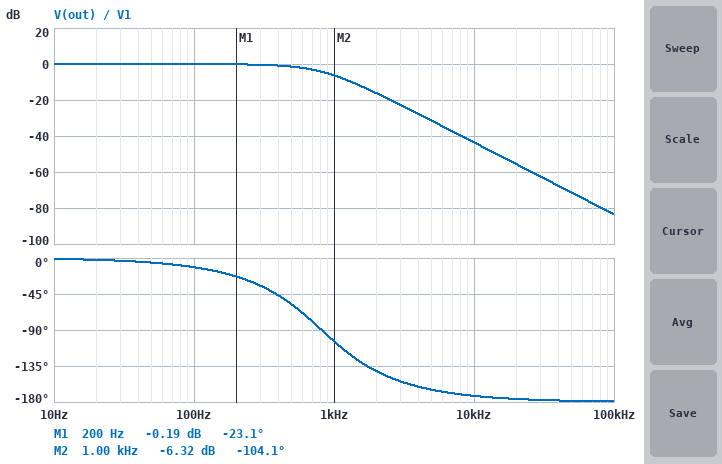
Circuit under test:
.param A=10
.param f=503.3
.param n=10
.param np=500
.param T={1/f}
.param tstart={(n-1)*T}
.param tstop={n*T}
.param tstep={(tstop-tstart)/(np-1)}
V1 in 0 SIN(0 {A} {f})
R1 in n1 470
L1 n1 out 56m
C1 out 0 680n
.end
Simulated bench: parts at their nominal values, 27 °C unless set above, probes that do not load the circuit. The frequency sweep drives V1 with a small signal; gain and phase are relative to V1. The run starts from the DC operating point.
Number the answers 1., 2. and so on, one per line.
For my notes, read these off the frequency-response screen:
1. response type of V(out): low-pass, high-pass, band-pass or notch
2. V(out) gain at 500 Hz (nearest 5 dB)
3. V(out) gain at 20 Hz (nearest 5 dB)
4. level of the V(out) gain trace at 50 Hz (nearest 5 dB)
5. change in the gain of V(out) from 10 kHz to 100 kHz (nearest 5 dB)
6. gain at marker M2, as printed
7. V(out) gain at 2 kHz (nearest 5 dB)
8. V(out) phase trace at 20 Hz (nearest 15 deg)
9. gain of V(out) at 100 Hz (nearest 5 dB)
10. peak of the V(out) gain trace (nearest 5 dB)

1. low-pass
2. 0 dB
3. 0 dB
4. 0 dB
5. -40 dB
6. -6.32 dB
7. -15 dB
8. 0 deg
9. 0 dB
10. 0 dB
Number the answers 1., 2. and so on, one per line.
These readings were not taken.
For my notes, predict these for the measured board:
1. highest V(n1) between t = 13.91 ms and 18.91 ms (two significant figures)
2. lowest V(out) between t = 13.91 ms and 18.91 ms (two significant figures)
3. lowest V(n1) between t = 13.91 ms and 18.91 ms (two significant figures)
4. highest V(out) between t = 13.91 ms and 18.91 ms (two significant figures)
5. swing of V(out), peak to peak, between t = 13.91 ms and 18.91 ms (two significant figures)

1. 5.2 V
2. -8.4 V
3. -5.2 V
4. 8.4 V
5. 17 V
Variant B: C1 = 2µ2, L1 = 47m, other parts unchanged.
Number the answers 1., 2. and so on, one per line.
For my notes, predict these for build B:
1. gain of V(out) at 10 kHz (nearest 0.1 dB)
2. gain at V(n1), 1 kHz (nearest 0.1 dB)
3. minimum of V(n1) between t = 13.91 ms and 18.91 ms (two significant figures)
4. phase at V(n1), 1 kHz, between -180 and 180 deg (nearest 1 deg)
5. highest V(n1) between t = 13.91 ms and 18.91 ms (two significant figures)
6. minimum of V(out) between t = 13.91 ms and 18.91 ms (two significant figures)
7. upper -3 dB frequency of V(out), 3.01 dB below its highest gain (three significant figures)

1. -52.3 dB
2. -7.4 dB
3. -100 mV
4. 65 deg
5. 100 mV
6. -3.1 V
7. 170 Hz
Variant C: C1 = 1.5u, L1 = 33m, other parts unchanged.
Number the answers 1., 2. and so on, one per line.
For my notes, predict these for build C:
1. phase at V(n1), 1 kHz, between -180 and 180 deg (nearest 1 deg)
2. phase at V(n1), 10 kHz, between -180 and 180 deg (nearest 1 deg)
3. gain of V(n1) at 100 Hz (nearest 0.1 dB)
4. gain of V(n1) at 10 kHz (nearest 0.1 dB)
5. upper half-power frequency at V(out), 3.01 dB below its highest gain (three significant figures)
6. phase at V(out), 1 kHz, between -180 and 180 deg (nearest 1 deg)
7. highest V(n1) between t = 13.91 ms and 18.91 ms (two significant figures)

1. 78 deg
2. 13 deg
3. -0.8 dB
4. -0.2 dB
5. 250 Hz
6. -102 deg
7. 2.2 V
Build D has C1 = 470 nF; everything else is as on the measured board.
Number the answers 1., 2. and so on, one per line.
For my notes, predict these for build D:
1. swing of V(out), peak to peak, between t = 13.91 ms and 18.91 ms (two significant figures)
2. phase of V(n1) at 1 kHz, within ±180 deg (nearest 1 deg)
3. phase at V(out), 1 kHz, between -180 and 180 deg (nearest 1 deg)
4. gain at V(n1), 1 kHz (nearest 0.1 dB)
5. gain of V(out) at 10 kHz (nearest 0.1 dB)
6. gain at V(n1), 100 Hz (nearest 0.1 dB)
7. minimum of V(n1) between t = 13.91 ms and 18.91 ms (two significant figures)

1. 20 V
2. 88 deg
3. -92 deg
4. -31.0 dB
5. -40.3 dB
6. -0.1 dB
7. -7.3 V
